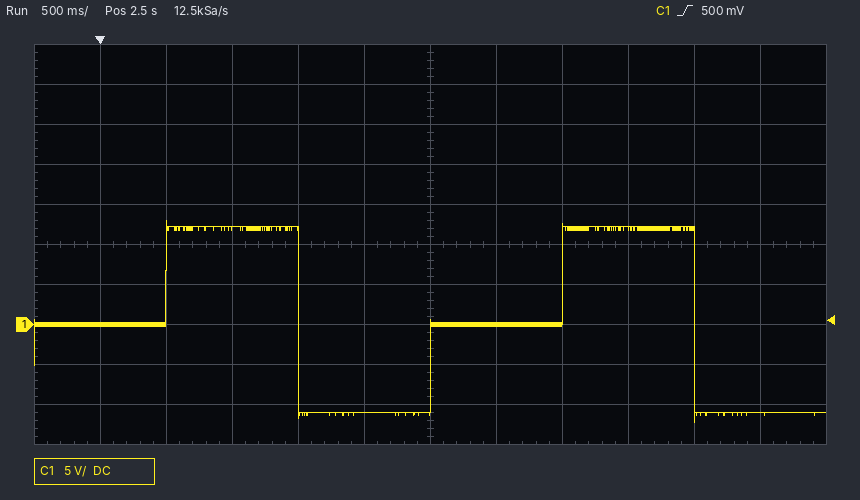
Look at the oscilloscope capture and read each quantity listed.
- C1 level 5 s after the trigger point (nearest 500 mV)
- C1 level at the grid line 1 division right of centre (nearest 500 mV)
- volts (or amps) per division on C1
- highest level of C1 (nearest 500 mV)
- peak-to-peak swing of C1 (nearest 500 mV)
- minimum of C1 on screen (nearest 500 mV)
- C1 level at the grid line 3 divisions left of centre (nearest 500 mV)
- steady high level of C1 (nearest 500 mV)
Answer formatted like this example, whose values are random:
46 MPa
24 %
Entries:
-11.0 V
0.0 V
5 V
13.0 V
25.0 V
-12.0 V
12.0 V
12.0 V
